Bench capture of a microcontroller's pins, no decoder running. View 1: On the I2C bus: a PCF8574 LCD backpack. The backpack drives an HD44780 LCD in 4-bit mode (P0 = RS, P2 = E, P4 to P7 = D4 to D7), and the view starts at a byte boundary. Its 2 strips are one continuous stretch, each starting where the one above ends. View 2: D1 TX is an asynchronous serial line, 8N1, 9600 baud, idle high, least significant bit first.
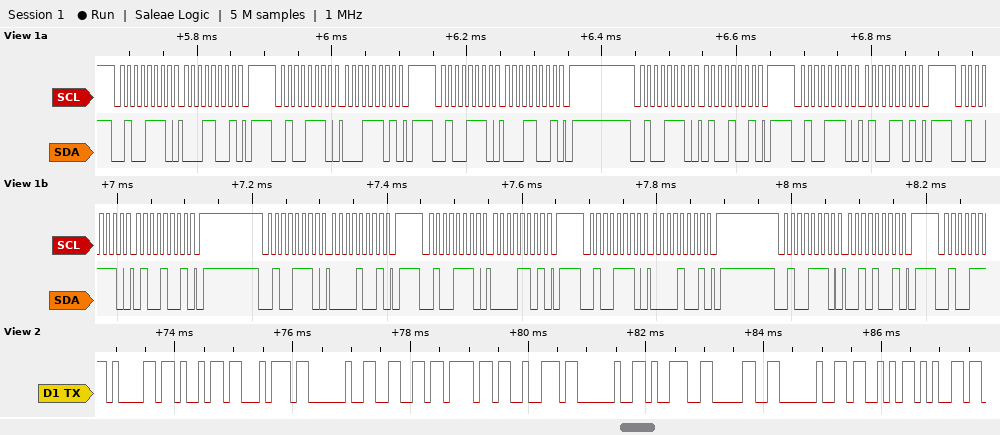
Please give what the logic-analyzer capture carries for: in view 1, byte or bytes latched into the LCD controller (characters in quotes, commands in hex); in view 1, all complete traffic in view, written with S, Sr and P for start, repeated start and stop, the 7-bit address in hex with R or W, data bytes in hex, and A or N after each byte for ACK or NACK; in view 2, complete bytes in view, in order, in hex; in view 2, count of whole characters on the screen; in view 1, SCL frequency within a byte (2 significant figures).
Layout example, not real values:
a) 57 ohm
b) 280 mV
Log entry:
a) data 0x14
b) S 27W A 19 A P S 27W A 1D A P S 27W A 19 A P S 27W A 49 A P S 27W A 4D A P S 27W A 49 A P S 27W A 09 A P S 27W A 0D A P S 27W A 09 A P S 27W A 29 A P
c) 0x61 0x69 0x74 0x20 0x66 0x6F 0x72 0x20 0x39 0x30 0x20 0x53 0x65
d) 13
e) 100 kHz
